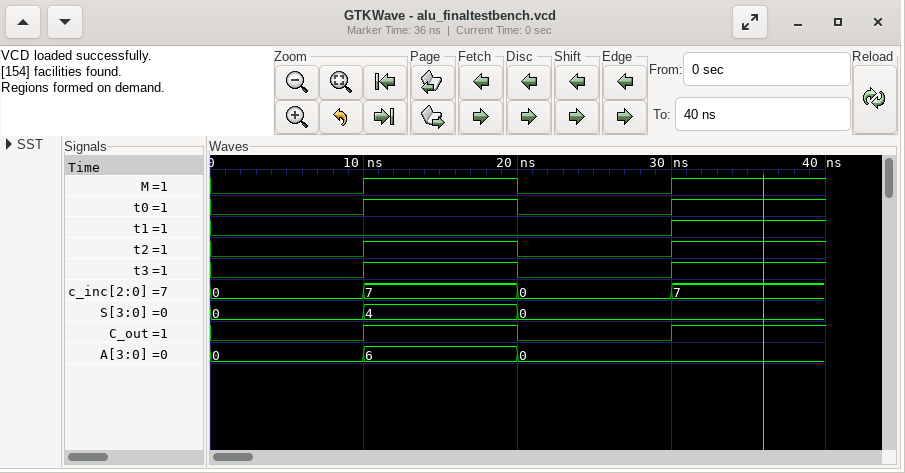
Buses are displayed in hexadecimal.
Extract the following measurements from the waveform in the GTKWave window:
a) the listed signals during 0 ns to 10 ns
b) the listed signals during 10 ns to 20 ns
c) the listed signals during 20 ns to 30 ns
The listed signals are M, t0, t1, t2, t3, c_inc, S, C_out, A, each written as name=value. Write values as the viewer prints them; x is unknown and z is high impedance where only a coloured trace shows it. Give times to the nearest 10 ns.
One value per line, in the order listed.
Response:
M=0, t0=0, t1=0, t2=0, t3=0, c_inc=0, S=0, C_out=0, A=0
M=1, t0=1, t1=0, t2=1, t3=1, c_inc=7, S=4, C_out=1, A=6
M=0, t0=0, t1=0, t2=0, t3=0, c_inc=0, S=0, C_out=0, A=0
